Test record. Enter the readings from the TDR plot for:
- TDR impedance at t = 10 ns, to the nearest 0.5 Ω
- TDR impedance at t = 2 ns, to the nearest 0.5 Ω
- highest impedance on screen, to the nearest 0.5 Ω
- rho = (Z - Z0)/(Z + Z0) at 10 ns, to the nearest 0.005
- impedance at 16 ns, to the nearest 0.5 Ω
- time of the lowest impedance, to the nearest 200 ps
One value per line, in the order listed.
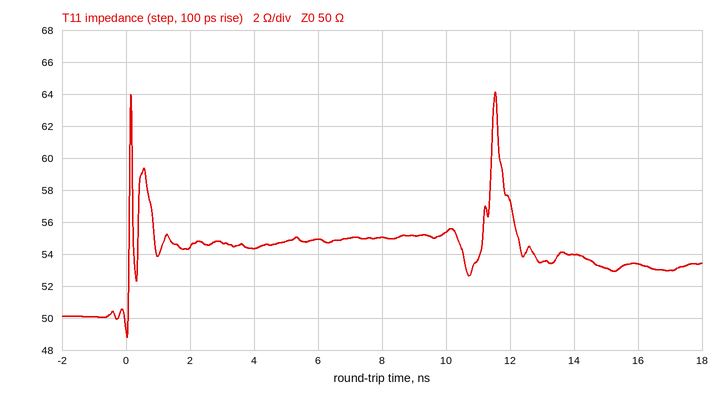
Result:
55.5 Ω
54.5 Ω
64.0 Ω
+0.050
53.5 Ω
0.0 ns
